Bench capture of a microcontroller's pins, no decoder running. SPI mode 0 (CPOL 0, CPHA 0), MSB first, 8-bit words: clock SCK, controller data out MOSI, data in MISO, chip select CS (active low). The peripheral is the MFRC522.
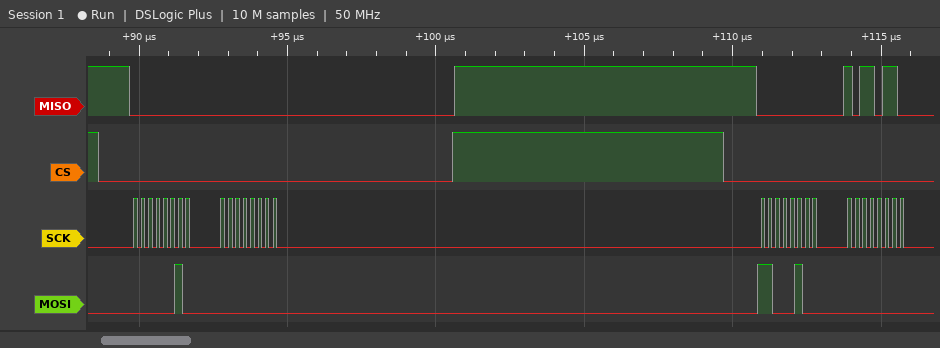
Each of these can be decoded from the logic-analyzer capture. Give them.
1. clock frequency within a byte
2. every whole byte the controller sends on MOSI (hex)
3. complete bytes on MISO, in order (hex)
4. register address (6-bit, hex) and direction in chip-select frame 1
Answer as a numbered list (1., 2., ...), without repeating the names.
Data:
1. 4 MHz
2. 02 00 C4 00
3. 00 00 00 B6
4. 0x01 write
